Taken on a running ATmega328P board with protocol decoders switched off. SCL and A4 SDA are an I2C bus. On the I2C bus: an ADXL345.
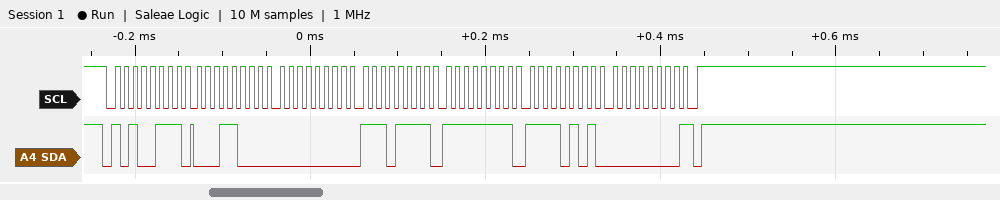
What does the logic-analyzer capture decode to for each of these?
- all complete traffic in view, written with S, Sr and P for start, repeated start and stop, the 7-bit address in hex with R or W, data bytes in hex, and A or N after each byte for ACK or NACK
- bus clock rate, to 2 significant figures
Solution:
S 53R A 18 A 00 A EF A FF A F5 A 00 N P
100 kHz
